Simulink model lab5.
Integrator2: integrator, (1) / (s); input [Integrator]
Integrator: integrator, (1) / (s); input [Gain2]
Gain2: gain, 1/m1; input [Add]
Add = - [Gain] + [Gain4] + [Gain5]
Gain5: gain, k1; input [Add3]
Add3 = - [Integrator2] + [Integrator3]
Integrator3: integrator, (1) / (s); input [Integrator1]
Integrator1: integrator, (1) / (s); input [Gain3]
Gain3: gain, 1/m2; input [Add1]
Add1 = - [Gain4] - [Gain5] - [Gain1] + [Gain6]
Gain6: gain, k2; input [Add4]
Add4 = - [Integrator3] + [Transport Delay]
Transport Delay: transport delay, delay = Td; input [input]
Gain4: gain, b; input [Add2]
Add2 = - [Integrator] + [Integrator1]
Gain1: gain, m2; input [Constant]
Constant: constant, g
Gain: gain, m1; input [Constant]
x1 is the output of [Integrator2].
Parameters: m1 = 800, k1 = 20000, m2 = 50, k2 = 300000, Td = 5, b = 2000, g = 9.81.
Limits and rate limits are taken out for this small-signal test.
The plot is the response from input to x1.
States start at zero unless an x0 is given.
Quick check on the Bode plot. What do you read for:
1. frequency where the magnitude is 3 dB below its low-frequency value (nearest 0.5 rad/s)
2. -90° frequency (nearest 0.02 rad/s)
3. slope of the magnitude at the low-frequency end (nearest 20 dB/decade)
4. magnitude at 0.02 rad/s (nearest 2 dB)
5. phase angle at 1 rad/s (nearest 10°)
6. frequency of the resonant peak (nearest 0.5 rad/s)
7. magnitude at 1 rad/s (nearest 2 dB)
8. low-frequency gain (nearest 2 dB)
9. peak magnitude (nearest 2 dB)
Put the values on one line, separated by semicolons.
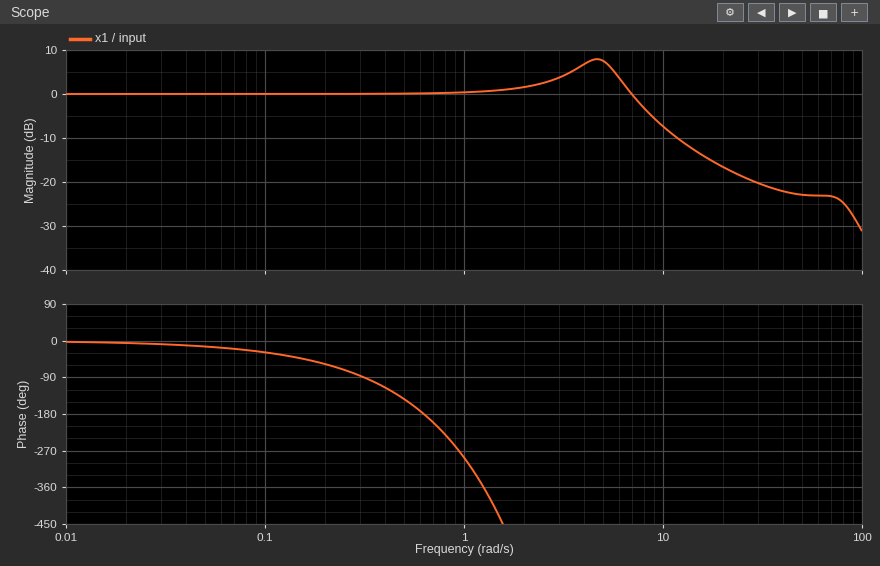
8.0 rad/s; 0.32 rad/s; 0 dB/decade; 0 dB; -290°; 4.5 rad/s; 0 dB; 0 dB; 8 dB
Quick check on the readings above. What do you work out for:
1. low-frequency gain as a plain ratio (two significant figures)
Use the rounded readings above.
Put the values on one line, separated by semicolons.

1.0
